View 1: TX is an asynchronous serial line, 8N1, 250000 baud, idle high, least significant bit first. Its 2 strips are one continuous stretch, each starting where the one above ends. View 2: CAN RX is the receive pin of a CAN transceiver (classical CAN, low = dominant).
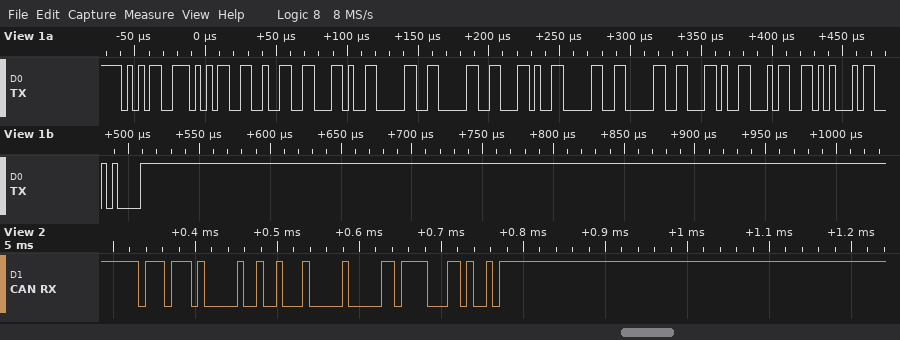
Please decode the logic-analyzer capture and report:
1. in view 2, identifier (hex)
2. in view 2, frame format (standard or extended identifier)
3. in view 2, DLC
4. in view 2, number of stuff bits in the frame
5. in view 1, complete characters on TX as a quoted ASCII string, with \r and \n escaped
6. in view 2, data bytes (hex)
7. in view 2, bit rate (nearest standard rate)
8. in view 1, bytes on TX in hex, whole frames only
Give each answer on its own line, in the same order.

0x774
standard
2
3
"552,00,00,4E\n"
44 00
125 kbit/s
35 35 32 2C 30 30 2C 30 30 2C 34 45 0A
